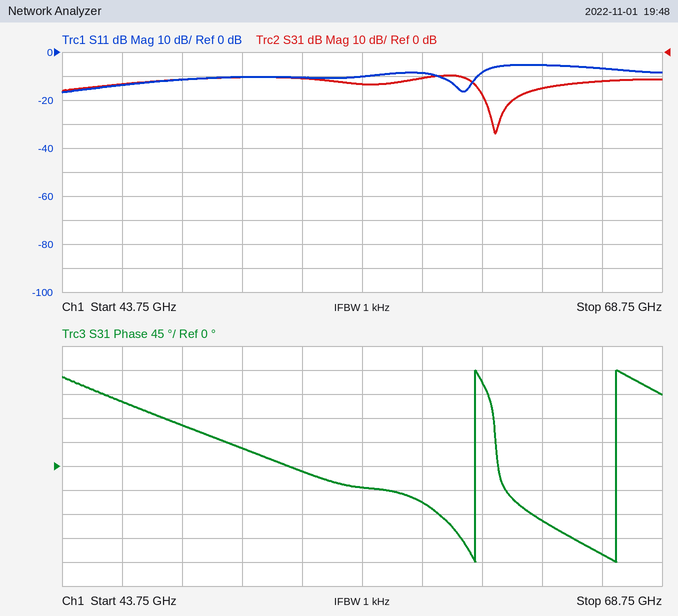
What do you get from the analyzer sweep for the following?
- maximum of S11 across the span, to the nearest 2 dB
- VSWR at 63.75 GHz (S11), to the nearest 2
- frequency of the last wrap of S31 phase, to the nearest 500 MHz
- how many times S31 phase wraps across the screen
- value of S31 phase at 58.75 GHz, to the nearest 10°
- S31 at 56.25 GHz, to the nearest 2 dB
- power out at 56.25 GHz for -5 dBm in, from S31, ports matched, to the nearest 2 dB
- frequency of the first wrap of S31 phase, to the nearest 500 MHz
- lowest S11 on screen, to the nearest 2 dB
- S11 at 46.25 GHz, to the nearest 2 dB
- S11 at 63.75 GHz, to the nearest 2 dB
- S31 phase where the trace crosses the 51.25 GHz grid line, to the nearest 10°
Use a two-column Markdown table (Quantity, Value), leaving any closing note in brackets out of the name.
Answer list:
| Quantity | Value |
|---|---|
| maximum of S11 across the span, to the nearest 2 dB | -6 dB |
| VSWR at 63.75 GHz (S11), to the nearest 2 | 4 |
| frequency of the last wrap of S31 phase, to the nearest 500 MHz | 67.0 GHz |
| how many times S31 phase wraps across the screen | 2 |
| value of S31 phase at 58.75 GHz, to the nearest 10° | -70° |
| S31 at 56.25 GHz, to the nearest 2 dB | -14 dB |
| power out at 56.25 GHz for -5 dBm in, from S31, ports matched, to the nearest 2 dB | -18 dBm |
| frequency of the first wrap of S31 phase, to the nearest 500 MHz | 61.0 GHz |
| lowest S11 on screen, to the nearest 2 dB | -16 dB |
| S11 at 46.25 GHz, to the nearest 2 dB | -14 dB |
| S11 at 63.75 GHz, to the nearest 2 dB | -6 dB |
| S31 phase where the trace crosses the 51.25 GHz grid line, to the nearest 10° | 30° |
